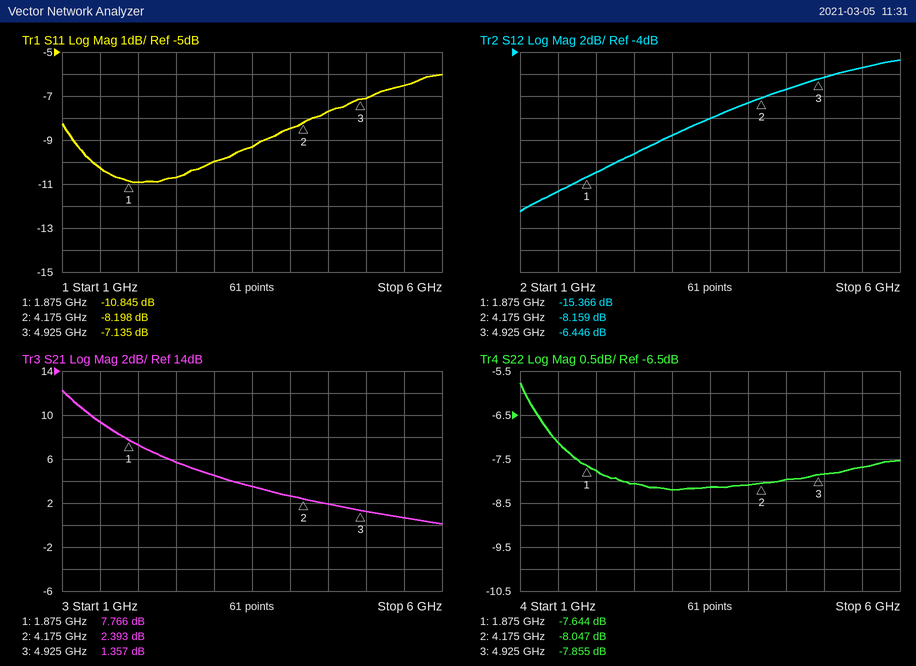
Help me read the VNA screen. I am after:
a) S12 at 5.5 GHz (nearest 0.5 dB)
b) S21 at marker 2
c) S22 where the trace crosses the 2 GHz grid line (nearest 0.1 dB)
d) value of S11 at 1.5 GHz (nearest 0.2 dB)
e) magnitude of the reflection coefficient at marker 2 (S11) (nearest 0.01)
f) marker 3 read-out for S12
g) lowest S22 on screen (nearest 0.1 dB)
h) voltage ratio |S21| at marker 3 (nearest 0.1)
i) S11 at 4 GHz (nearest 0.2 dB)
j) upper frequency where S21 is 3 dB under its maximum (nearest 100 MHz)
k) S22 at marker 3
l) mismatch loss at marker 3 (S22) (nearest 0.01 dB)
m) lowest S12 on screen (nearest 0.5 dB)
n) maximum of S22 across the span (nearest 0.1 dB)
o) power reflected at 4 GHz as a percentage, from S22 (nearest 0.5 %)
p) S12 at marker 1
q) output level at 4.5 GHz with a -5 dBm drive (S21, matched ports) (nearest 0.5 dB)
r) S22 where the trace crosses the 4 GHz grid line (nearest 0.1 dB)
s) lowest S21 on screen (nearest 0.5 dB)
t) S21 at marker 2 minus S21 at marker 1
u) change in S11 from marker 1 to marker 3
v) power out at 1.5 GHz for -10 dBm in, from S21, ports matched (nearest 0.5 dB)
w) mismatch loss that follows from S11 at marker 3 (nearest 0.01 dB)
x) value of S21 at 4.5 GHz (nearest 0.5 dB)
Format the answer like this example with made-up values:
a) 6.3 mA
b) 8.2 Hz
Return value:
a) -5.5 dB
b) 2.393 dB
c) -7.8 dB
d) -10.2 dB
e) 0.39
f) -6.446 dB
g) -8.2 dB
h) 1.2
i) -8.4 dB
j) 1.5 GHz
k) -7.855 dB
l) 0.78 dB
m) -18.5 dB
n) -5.8 dB
o) 15.5 %
p) -15.366 dB
q) -3.0 dBm
r) -8.1 dB
s) 0.0 dB
t) -5.373 dB
u) 3.710 dB
v) -0.5 dBm
w) 0.93 dB
x) 2.0 dB
